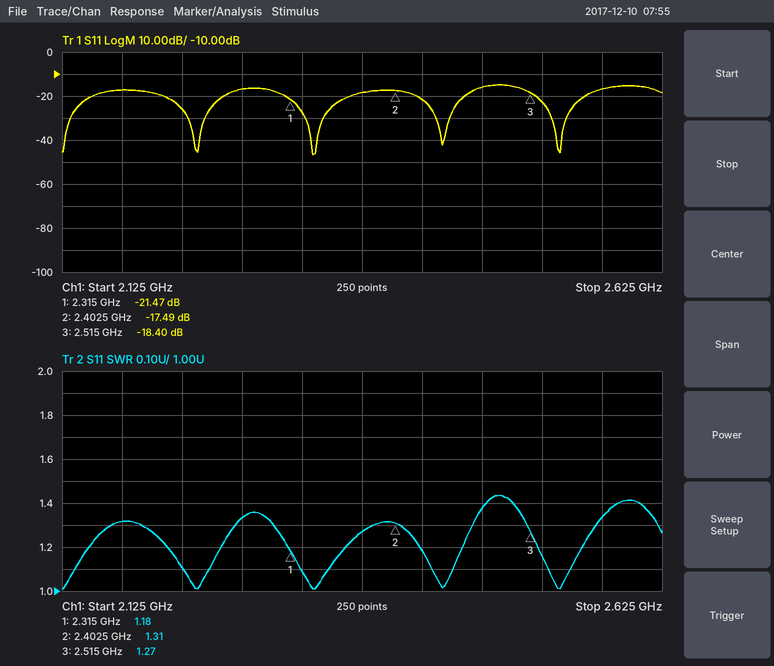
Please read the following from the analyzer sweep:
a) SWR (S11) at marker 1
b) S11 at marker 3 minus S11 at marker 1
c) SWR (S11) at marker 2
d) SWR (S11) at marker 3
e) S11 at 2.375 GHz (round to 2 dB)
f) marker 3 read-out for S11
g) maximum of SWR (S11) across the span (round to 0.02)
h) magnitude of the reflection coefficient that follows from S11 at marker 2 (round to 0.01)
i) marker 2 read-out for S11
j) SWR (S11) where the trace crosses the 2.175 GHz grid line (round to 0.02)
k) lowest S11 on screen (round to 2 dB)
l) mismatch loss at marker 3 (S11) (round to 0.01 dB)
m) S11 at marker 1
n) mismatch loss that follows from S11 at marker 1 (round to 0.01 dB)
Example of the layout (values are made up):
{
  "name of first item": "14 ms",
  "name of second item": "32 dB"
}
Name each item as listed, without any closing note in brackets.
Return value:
{
  "SWR (S11) at marker 1": "1.18",
  "S11 at marker 3 minus S11 at marker 1": "3.07 dB",
  "SWR (S11) at marker 2": "1.31",
  "SWR (S11) at marker 3": "1.27",
  "S11 at 2.375 GHz": "-18 dB",
  "marker 3 read-out for S11": "-18.40 dB",
  "maximum of SWR (S11) across the span": "1.44",
  "magnitude of the reflection coefficient that follows from S11 at marker 2": "0.13",
  "marker 2 read-out for S11": "-17.49 dB",
  "SWR (S11) where the trace crosses the 2.175 GHz grid line": "1.32",
  "lowest S11 on screen": "-46 dB",
  "mismatch loss at marker 3 (S11)": "0.06 dB",
  "S11 at marker 1": "-21.47 dB",
  "mismatch loss that follows from S11 at marker 1": "0.03 dB"
}
